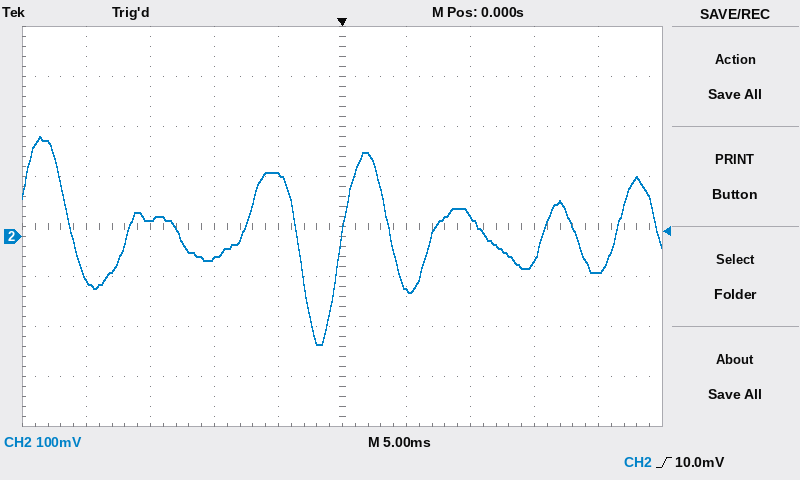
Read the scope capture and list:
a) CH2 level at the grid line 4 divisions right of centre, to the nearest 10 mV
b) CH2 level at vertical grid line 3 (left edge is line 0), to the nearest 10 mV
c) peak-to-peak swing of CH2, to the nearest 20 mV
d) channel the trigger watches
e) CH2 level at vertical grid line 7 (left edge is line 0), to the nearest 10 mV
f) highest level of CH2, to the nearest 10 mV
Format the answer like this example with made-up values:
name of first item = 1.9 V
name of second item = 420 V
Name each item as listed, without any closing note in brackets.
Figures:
CH2 level at the grid line 4 divisions right of centre, to the nearest 10 mV = -70 mV
CH2 level at vertical grid line 3 (left edge is line 0), to the nearest 10 mV = -40 mV
peak-to-peak swing of CH2, to the nearest 20 mV = 420 mV
channel the trigger watches = CH2
CH2 level at vertical grid line 7 (left edge is line 0), to the nearest 10 mV = 40 mV
highest level of CH2, to the nearest 10 mV = 200 mV
